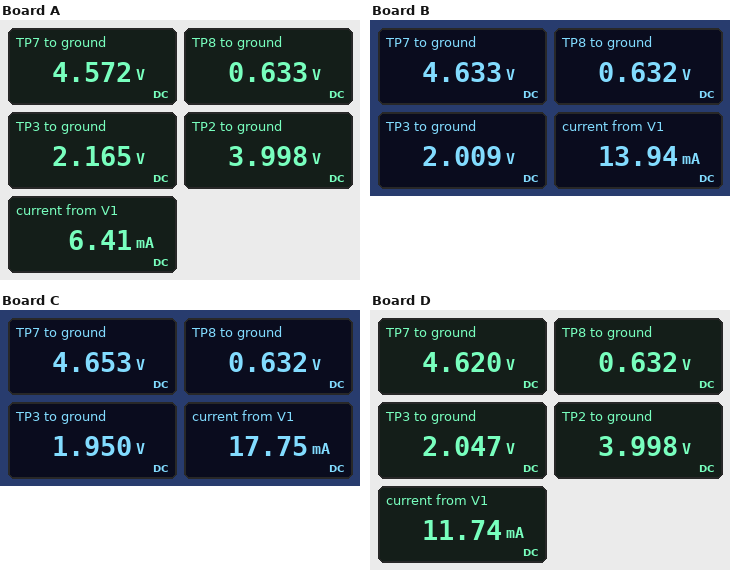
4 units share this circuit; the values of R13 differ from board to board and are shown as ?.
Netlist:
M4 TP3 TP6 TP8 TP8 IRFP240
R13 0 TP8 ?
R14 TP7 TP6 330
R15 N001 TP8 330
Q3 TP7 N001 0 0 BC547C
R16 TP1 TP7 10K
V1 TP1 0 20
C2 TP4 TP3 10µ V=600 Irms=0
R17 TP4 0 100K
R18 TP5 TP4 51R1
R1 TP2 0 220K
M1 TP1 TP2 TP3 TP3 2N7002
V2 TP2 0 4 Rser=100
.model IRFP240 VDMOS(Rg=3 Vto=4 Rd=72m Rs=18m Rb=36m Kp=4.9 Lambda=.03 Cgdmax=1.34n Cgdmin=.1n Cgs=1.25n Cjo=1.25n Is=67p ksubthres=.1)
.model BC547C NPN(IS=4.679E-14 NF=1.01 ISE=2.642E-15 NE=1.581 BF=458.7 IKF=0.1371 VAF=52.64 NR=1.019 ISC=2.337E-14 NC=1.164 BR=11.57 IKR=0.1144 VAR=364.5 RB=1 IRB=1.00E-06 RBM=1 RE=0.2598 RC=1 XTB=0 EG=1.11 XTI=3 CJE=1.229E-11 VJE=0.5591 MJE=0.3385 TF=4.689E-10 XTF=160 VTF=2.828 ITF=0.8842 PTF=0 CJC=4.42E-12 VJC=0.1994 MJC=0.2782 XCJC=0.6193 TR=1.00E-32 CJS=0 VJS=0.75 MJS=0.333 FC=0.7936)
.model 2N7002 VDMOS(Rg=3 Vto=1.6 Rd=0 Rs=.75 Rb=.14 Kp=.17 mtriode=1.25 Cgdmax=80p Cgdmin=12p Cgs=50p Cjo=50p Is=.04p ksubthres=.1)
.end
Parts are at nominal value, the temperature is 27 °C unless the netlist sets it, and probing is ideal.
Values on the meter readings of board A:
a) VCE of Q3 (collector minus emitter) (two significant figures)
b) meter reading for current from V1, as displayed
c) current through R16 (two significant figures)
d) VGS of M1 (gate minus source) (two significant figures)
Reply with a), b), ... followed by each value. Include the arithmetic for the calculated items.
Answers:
a) 4.572 V = 4.6 V
b) 6.41 mA
c) (20 V - 4.572 V) / 10 kΩ = 1.5 mA
d) 3.998 V - 2.165 V = 1.8 V
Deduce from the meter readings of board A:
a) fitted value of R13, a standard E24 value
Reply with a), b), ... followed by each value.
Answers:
a) 130 Ω
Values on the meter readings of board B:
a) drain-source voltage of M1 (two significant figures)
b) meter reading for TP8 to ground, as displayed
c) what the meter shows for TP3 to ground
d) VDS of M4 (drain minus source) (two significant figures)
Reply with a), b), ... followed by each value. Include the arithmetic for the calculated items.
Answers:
a) 20 V - 2.009 V = 18 V
b) 0.632 V
c) 2.009 V
d) 2.009 V - 632 mV = 1.4 V
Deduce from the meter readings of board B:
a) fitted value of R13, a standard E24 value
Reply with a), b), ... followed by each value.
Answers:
a) 51 Ω
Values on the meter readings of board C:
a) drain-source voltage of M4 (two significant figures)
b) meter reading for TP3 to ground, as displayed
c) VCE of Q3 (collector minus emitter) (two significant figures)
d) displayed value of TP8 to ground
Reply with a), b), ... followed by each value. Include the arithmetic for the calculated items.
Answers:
a) 1.95 V - 632 mV = 1.3 V
b) 1.950 V
c) 4.653 V = 4.7 V
d) 0.632 V
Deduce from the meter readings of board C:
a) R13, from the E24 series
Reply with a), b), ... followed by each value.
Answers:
a) 39 Ω
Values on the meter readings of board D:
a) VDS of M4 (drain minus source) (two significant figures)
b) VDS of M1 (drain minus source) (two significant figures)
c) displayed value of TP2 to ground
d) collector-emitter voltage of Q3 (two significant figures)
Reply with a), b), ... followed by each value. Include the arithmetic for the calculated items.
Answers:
a) 2.047 V - 632 mV = 1.4 V
b) 20 V - 2.047 V = 18 V
c) 3.998 V
d) 4.62 V = 4.6 V
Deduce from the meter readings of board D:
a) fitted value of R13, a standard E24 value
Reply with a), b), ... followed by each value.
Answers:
a) 62 Ω
